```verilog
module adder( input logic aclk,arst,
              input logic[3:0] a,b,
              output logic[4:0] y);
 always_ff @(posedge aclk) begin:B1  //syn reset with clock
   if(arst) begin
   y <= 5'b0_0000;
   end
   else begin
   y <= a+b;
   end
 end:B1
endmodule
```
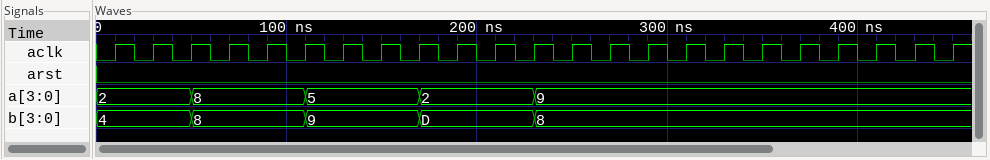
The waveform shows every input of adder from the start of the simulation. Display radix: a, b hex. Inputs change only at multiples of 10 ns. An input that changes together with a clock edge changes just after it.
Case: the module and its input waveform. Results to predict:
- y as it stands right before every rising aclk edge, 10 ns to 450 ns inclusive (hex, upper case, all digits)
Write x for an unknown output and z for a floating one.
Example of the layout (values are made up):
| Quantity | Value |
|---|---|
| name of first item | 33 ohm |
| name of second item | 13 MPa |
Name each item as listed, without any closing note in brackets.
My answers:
| Quantity | Value |
|---|---|
| y as it stands right before every rising aclk edge, 10 ns to 450 ns inclusive | x, 06, 06, 06, 10, 10, 10, 0E, 0E, 0E, 0F, 0F, 0F, 11, 11, 11, 11, 11, 11, 11, 11, 11, 11 |
